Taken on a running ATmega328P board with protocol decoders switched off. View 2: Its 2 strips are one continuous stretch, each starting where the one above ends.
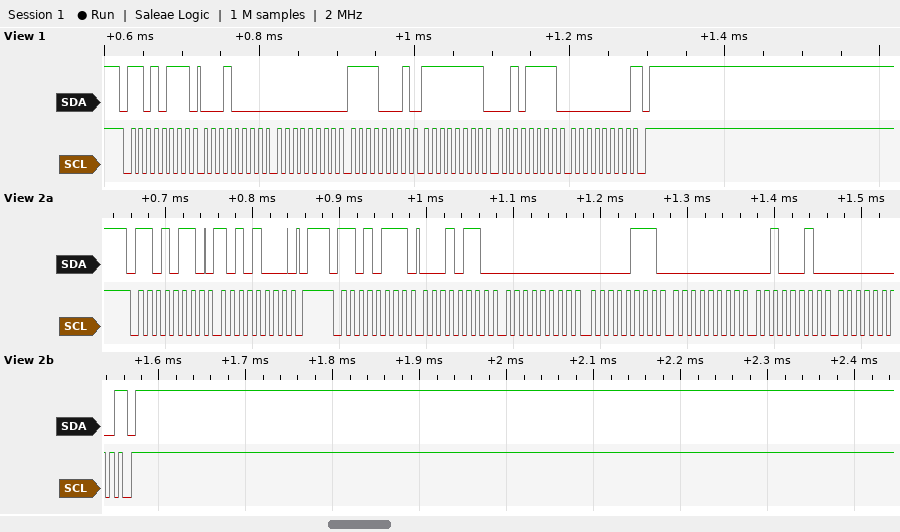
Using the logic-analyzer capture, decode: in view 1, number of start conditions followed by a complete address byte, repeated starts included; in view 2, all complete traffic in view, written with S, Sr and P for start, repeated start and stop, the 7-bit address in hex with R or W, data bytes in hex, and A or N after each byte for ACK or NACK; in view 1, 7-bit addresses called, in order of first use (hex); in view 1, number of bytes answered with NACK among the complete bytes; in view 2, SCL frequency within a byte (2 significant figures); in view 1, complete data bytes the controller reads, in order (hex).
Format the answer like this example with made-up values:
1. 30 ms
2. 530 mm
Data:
1. 1
2. S 6BW A A8 A P S 6BR A 16 A 00 A 07 A 00 A 22 A 00 N P
3. 0x6B
4. 1
5. 100 kHz
6. 10 00 F1 FF 2F 00
